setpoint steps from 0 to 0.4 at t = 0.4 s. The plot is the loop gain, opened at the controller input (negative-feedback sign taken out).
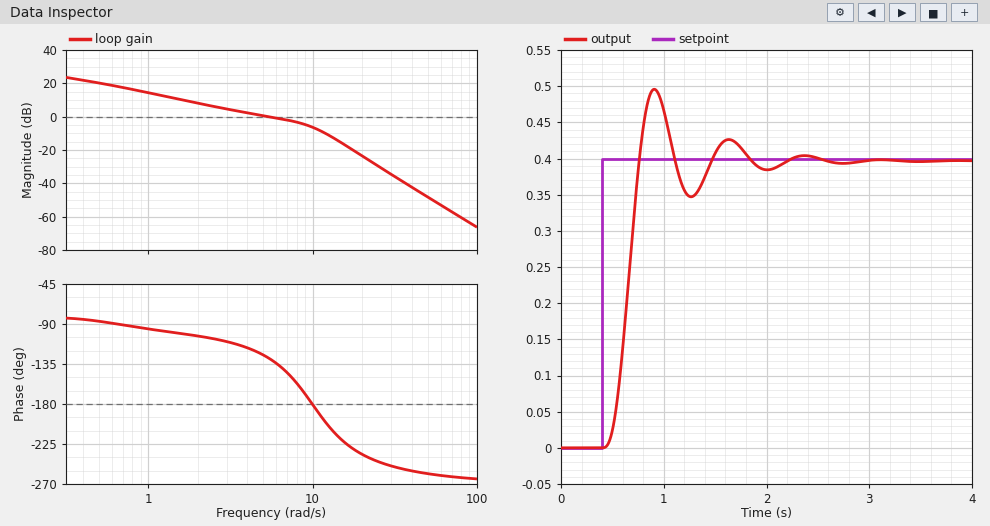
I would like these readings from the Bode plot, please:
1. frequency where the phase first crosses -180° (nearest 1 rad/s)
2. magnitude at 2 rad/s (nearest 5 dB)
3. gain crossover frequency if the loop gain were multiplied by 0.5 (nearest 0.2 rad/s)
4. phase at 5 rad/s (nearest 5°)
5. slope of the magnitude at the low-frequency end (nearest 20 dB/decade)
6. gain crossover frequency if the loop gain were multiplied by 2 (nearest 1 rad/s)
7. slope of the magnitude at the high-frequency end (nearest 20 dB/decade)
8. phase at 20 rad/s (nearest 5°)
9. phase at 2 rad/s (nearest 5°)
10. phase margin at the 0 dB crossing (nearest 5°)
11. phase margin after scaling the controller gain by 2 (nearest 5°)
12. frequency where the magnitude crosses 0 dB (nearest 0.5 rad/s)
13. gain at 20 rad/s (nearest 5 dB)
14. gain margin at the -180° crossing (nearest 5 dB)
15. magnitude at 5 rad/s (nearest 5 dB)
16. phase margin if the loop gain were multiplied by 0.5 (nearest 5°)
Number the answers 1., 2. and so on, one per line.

1. 10 rad/s
2. 10 dB
3. 2.6 rad/s
4. -125°
5. -20 dB/decade
6. 10 rad/s
7. -60 dB/decade
8. -235°
9. -105°
10. 50°
11. 0°
12. 5.5 rad/s
13. -25 dB
14. 5 dB
15. 0 dB
16. 75°
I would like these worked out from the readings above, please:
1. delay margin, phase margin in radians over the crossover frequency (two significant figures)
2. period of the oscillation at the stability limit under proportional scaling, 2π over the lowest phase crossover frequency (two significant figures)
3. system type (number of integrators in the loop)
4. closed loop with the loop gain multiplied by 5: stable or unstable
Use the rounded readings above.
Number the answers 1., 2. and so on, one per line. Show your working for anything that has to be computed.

1. 50 × π / 180 / 5.5 = 0.16 s
2. 2π / 10 = 0.63 s
3. 1
4. unstable
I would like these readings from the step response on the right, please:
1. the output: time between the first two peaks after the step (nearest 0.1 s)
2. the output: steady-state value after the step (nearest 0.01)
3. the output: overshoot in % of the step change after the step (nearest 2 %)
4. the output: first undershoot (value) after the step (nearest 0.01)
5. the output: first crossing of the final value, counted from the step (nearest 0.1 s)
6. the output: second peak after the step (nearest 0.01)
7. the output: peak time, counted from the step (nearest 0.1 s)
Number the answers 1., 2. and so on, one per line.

1. 0.7 s
2. 0.40
3. 24 %
4. 0.35
5. 0.4 s
6. 0.43
7. 0.5 s
